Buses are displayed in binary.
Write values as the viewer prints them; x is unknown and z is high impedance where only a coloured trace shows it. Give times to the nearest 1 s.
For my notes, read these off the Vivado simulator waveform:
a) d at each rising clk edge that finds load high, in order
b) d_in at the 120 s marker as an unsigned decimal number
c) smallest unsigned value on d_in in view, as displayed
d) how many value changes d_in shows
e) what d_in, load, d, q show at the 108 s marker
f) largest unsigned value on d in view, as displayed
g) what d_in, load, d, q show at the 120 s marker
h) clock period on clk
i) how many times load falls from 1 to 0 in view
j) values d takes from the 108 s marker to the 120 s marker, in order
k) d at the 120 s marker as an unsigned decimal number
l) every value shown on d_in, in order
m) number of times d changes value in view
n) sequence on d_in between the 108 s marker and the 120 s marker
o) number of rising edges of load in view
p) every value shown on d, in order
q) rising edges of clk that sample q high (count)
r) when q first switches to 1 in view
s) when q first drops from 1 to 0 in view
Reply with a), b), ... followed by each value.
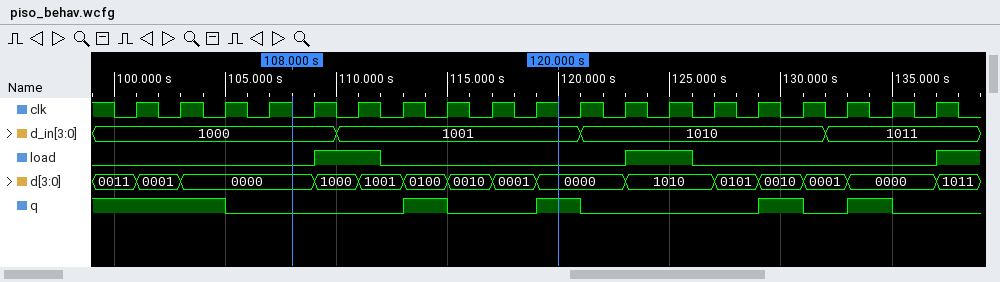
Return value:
a) 1000, 1010
b) 9
c) 1000
d) 3
e) d_in=1000, load=0, d=0000, q=0
f) 1011
g) d_in=1001, load=0, d=0000, q=1
h) 2 s
i) 2
j) 0000, 1000, 1001, 0100, 0010, 0001, 0000
k) 0
l) 1000, 1001, 1010, 1011
m) 14
n) 1000, 1001
o) 3
p) 0011, 0001, 0000, 1000, 1001, 0100, 0010, 0001, 0000, 1010, 0101, 0010, 0001, 0000, 1011
q) 7
r) 113 s
s) 105 s
